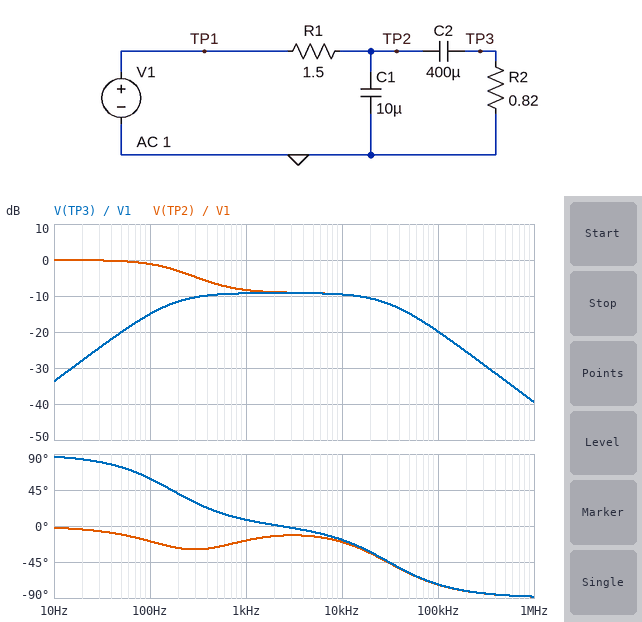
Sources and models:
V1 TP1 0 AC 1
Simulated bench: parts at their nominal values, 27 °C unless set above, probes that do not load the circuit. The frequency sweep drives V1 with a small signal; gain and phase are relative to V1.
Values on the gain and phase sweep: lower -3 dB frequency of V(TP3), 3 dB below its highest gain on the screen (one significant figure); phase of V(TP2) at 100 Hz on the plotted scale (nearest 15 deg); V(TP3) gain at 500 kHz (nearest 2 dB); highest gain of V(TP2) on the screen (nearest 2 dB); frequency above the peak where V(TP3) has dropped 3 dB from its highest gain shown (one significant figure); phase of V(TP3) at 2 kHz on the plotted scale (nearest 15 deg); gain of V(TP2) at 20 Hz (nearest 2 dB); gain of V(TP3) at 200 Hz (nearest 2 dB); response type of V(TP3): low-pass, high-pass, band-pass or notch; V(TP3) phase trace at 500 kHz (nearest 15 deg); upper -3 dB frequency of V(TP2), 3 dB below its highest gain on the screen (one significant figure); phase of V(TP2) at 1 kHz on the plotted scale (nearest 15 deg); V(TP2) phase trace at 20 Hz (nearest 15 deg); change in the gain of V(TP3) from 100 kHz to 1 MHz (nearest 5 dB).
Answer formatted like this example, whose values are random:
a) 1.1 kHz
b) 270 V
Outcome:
a) 200 Hz
b) -15 deg
c) -34 dB
d) 0 dB
e) 30 kHz
f) 0 deg
g) 0 dB
h) -12 dB
i) band-pass
j) -90 deg
k) 200 Hz
l) -15 deg
m) 0 deg
n) -20 dB
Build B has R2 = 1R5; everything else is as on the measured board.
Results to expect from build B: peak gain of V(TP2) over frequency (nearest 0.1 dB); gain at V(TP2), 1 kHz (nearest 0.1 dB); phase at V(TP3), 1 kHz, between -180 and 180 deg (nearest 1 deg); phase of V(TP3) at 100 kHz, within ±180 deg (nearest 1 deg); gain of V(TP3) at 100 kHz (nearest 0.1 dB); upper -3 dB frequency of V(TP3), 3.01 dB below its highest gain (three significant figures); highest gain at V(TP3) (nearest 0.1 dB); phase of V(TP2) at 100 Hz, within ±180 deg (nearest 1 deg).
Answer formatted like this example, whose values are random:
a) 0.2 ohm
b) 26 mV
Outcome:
a) 0 dB
b) -5.9 dB
c) 5 deg
d) -78 deg
e) -19.7 dB
f) 21.6 kHz
g) -6.1 dB
h) -17 deg
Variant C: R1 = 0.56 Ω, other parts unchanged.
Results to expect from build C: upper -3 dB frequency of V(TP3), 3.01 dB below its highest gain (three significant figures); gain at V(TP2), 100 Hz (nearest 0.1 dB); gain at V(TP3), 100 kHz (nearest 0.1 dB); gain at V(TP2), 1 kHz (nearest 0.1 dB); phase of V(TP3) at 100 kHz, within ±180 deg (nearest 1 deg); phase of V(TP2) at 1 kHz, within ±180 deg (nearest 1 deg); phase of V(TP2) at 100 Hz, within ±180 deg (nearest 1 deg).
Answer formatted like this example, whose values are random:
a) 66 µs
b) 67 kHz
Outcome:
a) 48.6 kHz
b) -0.3 dB
c) -11.8 dB
d) -4.0 dB
e) -64 deg
f) -11 deg
g) -8 deg
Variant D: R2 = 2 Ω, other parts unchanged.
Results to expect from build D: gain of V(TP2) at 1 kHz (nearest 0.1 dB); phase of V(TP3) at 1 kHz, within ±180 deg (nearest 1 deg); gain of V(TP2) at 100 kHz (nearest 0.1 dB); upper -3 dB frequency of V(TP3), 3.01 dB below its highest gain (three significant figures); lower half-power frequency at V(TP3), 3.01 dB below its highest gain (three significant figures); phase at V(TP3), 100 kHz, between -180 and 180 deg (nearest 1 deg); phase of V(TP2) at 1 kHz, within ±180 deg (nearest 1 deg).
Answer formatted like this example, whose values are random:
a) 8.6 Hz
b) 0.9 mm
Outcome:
a) -4.8 dB
b) 3 deg
c) -19.6 dB
d) 18.9 kHz
e) 112 Hz
f) -79 deg
g) -8 deg
